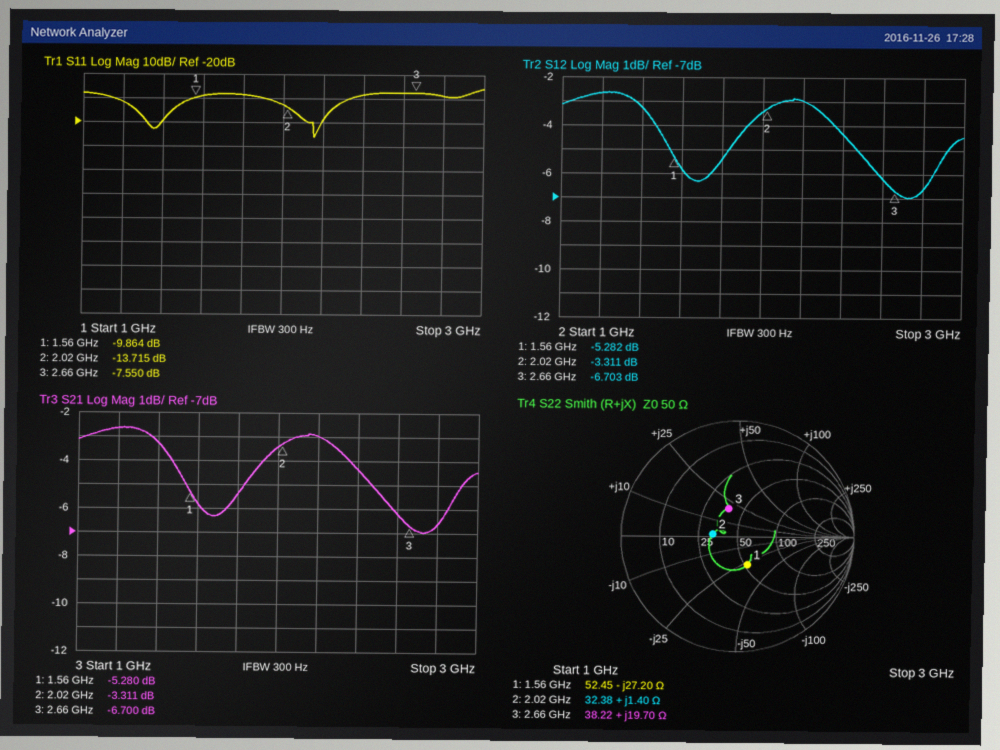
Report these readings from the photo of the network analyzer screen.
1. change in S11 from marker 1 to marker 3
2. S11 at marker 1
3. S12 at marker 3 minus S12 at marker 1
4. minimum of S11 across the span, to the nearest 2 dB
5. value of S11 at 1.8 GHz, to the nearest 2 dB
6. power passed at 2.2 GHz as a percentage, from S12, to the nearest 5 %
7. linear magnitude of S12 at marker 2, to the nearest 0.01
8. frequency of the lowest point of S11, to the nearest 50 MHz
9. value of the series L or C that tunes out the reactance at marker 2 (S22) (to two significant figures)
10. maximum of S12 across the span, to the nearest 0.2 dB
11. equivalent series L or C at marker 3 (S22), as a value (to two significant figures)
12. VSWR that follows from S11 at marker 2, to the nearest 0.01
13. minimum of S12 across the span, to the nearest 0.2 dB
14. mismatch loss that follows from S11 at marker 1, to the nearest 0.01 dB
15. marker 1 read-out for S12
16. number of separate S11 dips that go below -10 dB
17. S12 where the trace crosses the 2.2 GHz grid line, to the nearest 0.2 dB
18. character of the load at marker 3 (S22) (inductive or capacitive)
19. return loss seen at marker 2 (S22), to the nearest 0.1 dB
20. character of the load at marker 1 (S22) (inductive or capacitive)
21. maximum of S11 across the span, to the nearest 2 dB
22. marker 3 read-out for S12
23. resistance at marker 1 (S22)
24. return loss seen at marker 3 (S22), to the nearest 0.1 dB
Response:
2.314 dB
-9.864 dB
-1.421 dB
-26 dB
-8 dB
50 %
0.68
2.15 GHz
56 pF
-2.6 dB
1.2 nH
1.52
-7.0 dB
0.47 dB
-5.282 dB
2
-3.0 dB
inductive
13.4 dB
capacitive
-6 dB
-6.703 dB
52.45 Ω
11.9 dB
